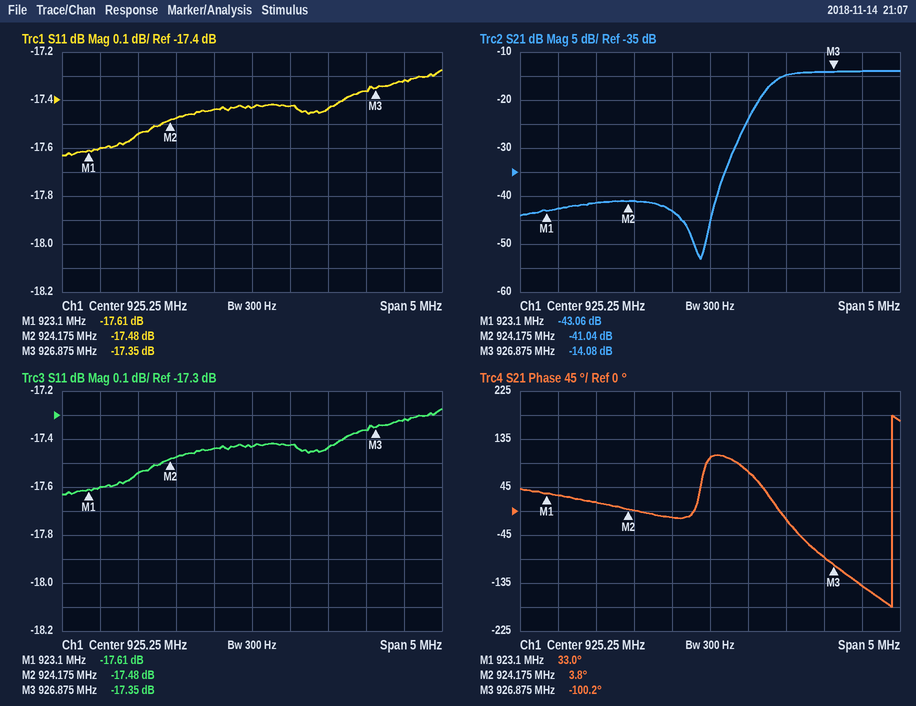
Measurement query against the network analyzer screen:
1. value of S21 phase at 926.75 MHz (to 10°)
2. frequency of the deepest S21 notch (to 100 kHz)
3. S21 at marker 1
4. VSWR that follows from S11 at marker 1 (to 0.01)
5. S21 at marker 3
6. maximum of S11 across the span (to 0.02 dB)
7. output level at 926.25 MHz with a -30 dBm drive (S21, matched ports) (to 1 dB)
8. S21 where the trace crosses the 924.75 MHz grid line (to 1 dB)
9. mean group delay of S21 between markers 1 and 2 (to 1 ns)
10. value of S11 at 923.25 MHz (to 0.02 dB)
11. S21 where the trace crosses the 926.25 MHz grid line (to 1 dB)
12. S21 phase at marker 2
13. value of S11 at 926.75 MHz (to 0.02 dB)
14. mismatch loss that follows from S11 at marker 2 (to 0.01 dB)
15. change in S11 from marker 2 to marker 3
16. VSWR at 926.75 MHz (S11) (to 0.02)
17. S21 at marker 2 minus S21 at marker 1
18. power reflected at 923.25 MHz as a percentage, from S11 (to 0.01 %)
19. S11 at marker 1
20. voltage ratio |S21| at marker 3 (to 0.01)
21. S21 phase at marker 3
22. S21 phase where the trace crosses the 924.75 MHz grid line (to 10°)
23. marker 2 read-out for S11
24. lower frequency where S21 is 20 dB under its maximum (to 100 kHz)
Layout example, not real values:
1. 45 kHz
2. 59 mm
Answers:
1. -90°
2. 925.1 MHz
3. -43.06 dB
4. 1.30
5. -14.08 dB
6. -17.28 dB
7. -45 dBm
8. -43 dB
9. 75 ns
10. -17.60 dB
11. -15 dB
12. 3.8°
13. -17.36 dB
14. 0.08 dB
15. 0.13 dB
16. 1.32
17. 2.02 dB
18. 1.74 %
19. -17.61 dB
20. 0.20
21. -100.2°
22. -10°
23. -17.48 dB
24. 925.5 MHz
